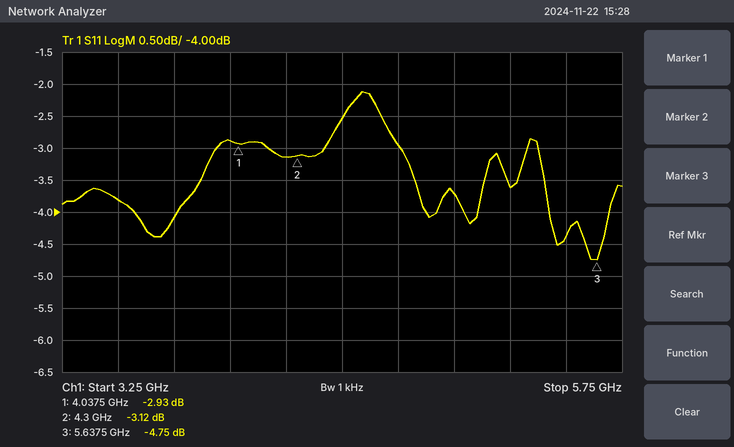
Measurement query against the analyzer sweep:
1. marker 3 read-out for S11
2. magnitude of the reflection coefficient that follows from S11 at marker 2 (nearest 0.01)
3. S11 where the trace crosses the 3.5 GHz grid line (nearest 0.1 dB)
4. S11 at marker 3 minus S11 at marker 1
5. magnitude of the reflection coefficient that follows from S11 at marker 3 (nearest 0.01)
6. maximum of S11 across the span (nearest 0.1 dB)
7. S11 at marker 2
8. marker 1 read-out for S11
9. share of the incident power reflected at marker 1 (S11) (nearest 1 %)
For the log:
-4.75 dB
0.70
-3.8 dB
-1.82 dB
0.58
-2.1 dB
-3.12 dB
-2.93 dB
51 %
